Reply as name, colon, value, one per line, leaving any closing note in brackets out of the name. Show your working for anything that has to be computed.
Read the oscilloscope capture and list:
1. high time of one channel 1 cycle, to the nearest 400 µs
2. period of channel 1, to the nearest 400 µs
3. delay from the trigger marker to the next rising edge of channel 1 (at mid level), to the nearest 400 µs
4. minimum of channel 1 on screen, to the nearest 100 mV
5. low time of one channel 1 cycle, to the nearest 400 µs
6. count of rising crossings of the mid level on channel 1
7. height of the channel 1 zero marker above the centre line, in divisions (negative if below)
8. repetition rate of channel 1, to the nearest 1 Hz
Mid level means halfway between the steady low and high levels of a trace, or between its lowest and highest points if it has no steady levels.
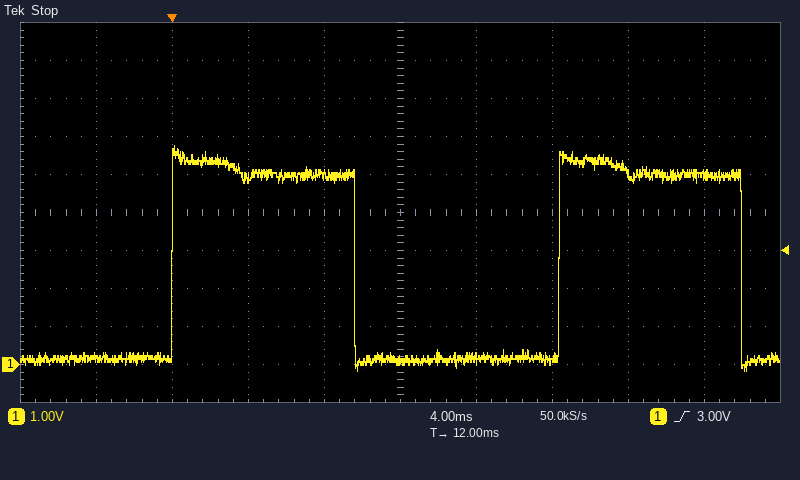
high time of one channel 1 cycle, to the nearest 400 µs: 9.6 ms
period of channel 1, to the nearest 400 µs: 20.4 ms
delay from the trigger marker to the next rising edge of channel 1 (at mid level), to the nearest 400 µs: 20.4 ms
minimum of channel 1 on screen, to the nearest 100 mV: -200 mV
low time of one channel 1 cycle, to the nearest 400 µs: 10.8 ms
count of rising crossings of the mid level on channel 1: 2
height of the channel 1 zero marker above the centre line, in divisions: -4.0 div
repetition rate of channel 1, to the nearest 1 Hz: 1 / 20.4 ms ≈ 49 Hz
